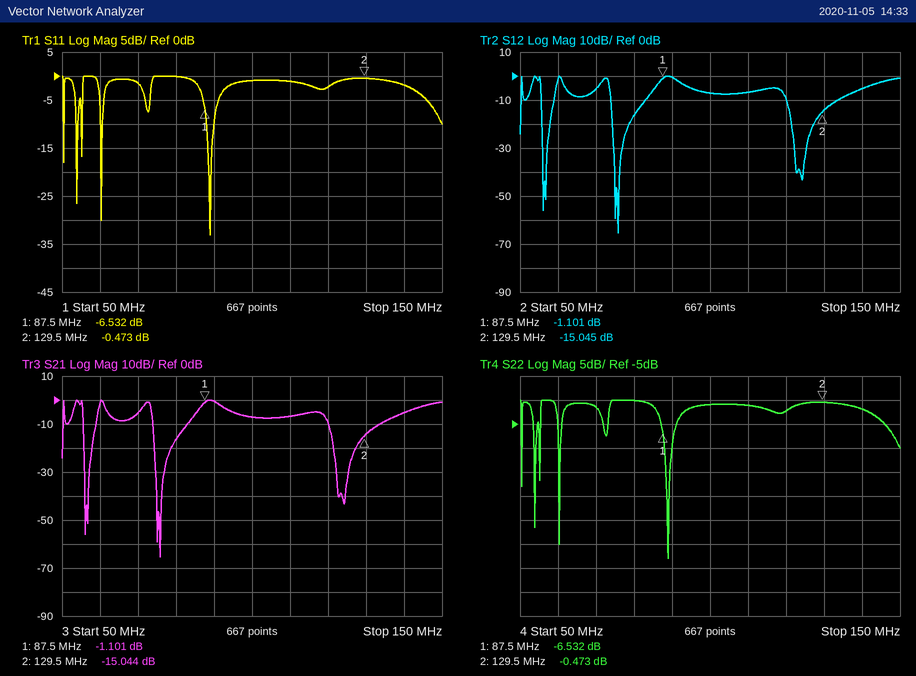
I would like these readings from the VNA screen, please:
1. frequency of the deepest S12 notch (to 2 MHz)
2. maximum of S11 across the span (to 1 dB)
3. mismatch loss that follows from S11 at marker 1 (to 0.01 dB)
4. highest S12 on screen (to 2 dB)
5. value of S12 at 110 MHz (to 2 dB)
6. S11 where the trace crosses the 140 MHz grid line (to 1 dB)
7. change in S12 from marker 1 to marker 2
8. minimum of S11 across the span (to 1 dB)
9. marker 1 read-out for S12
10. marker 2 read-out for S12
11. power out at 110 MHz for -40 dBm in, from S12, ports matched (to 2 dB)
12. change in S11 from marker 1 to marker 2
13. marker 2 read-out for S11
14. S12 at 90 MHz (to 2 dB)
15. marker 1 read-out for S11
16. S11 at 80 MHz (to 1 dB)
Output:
76 MHz
0 dB
1.09 dB
0 dB
-6 dB
-2 dB
-13.944 dB
-33 dB
-1.101 dB
-15.045 dB
-46 dBm
6.059 dB
-0.473 dB
0 dB
-6.532 dB
0 dB
